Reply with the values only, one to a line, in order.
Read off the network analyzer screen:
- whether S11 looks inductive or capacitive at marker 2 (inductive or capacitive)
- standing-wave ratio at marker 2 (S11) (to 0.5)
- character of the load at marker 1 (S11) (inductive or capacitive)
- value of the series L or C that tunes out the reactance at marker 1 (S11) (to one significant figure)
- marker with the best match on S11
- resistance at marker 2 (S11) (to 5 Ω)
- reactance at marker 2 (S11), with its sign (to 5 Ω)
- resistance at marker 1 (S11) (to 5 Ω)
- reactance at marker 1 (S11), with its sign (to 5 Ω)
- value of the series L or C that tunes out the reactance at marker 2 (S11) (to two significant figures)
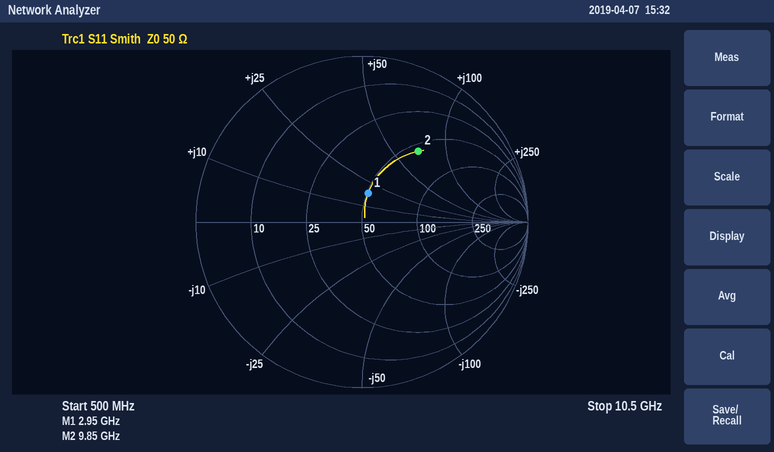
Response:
inductive
3.5
inductive
3 pF
marker 1
55 Ω
+70 Ω
50 Ω
+20 Ω
230 fF
